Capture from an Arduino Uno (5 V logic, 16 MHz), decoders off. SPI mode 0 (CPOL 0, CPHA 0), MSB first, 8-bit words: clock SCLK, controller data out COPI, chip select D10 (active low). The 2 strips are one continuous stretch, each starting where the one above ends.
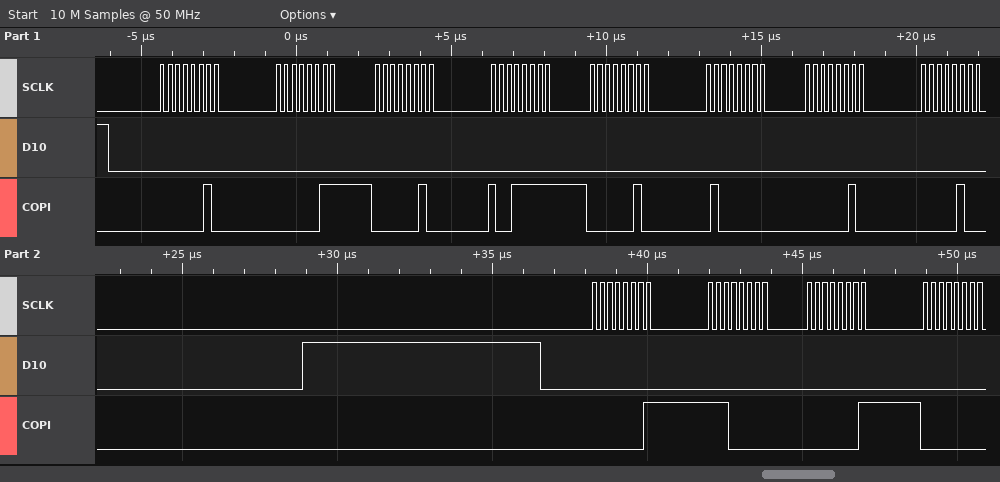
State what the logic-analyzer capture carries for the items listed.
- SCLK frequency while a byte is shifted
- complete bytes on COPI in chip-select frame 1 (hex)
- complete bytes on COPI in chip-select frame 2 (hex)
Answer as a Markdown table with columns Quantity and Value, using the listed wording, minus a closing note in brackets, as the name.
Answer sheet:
| Quantity | Value |
|---|---|
| SCLK frequency while a byte is shifted | 4 MHz |
| complete bytes on COPI in chip-select frame 1 | 02 03 02 9F 02 40 02 04 |
| complete bytes on COPI in chip-select frame 2 | 01 E0 01 00 |
